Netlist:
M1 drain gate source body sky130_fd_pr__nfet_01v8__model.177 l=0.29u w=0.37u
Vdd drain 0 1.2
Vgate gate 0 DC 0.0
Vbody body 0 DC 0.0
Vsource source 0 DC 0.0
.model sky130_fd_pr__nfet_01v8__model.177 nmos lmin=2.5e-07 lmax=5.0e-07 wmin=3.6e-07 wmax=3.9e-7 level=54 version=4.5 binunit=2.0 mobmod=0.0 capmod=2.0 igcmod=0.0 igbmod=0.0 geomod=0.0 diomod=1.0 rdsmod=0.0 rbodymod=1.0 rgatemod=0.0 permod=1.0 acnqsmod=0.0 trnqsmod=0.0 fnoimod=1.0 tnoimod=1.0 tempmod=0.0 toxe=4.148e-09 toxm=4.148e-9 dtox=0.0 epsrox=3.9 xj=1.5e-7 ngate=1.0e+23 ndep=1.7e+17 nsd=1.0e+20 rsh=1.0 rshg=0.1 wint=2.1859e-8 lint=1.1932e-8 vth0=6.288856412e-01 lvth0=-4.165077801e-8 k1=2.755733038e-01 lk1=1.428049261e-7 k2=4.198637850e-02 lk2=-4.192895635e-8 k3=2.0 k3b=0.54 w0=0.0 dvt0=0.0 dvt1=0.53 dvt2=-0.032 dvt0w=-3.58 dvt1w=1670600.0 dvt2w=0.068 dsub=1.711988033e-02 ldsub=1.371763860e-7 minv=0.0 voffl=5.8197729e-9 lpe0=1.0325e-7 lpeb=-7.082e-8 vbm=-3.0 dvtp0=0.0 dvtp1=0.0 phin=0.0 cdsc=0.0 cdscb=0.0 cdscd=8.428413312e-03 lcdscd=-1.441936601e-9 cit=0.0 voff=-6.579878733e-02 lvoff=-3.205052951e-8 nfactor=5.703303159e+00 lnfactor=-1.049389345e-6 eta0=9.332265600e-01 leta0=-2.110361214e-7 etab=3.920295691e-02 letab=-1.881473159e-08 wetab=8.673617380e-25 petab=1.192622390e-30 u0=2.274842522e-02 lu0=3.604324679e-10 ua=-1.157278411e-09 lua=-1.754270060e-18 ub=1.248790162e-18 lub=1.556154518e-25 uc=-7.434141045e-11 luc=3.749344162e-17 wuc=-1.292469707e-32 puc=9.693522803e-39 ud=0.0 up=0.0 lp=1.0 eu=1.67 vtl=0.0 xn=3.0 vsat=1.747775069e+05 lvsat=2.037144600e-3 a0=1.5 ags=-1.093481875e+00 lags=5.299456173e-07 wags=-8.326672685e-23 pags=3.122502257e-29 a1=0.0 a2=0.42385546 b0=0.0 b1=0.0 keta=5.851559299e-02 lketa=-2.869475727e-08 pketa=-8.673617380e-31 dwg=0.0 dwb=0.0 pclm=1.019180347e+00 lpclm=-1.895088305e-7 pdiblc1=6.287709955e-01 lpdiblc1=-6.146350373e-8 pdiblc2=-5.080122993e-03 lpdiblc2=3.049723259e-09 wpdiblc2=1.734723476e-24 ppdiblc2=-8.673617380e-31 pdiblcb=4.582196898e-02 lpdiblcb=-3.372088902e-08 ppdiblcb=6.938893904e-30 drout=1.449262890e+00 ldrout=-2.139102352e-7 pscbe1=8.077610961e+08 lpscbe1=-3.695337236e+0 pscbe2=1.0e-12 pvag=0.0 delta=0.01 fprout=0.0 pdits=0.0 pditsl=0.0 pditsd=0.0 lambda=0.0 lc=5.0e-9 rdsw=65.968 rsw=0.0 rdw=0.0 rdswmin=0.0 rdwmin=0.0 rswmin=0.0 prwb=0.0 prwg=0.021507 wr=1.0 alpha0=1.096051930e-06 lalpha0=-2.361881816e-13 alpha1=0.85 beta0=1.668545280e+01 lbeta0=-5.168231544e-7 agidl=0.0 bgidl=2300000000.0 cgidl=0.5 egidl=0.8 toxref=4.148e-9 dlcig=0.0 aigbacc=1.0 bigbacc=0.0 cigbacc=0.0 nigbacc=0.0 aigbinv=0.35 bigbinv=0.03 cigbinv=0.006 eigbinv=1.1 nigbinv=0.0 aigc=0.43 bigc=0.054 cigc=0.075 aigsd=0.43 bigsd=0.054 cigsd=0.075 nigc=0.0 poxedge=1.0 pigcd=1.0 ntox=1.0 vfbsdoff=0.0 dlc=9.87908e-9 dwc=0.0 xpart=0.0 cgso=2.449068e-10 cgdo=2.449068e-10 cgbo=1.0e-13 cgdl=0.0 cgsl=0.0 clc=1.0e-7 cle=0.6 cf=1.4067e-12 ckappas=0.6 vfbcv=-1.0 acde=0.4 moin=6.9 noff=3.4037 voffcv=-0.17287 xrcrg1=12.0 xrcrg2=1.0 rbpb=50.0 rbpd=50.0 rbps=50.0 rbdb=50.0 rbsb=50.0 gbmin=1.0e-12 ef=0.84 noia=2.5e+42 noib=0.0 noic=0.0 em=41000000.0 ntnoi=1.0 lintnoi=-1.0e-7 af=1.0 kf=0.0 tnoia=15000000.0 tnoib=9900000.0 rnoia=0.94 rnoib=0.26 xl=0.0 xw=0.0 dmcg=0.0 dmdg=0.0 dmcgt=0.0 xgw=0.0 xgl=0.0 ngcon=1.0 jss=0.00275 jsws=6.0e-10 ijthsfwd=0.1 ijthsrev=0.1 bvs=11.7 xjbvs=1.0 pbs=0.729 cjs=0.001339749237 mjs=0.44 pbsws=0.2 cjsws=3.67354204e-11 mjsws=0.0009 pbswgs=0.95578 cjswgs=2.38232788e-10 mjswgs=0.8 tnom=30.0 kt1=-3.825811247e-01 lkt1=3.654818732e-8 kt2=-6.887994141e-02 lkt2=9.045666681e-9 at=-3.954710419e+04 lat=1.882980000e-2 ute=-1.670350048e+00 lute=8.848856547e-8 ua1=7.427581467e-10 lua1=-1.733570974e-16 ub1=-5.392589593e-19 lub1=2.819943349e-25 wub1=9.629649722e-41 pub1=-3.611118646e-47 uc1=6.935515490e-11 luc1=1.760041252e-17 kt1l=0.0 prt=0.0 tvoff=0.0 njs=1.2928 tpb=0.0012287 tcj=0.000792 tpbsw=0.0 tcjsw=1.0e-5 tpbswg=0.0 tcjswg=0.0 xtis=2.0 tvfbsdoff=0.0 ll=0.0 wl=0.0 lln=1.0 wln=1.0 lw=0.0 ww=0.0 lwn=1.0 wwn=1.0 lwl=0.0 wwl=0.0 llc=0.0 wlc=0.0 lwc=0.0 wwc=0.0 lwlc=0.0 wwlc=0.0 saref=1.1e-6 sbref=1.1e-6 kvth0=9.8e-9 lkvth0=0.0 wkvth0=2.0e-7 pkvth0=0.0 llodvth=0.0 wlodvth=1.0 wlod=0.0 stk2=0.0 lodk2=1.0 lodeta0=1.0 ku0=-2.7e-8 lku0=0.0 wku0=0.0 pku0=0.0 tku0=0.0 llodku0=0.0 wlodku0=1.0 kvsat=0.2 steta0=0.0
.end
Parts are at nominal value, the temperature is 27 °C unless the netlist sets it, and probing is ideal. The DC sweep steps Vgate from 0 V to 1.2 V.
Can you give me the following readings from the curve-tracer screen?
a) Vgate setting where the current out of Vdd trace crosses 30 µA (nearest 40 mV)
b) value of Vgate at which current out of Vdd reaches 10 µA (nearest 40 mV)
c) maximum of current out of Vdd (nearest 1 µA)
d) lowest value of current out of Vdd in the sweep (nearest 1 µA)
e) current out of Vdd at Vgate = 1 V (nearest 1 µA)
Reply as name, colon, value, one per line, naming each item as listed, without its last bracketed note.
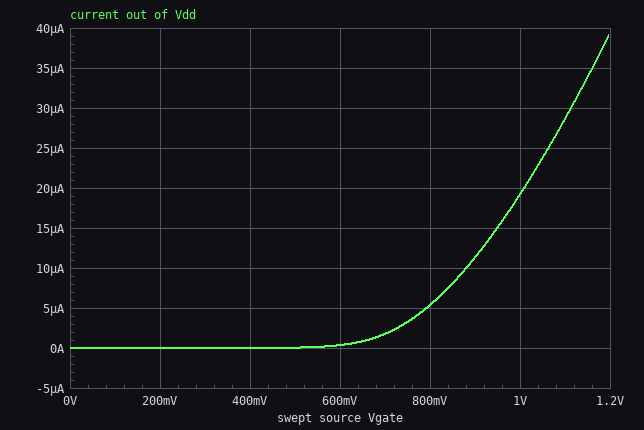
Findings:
Vgate setting where the current out of Vdd trace crosses 30 µA: 1.12 V
value of Vgate at which current out of Vdd reaches 10 µA: 880 mV
maximum of current out of Vdd: 39 µA
lowest value of current out of Vdd in the sweep: 0 A
current out of Vdd at Vgate = 1 V: 19 µA
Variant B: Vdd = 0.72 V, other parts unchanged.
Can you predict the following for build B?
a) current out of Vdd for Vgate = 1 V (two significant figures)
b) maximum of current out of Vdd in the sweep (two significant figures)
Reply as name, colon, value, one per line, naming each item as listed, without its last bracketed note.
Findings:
current out of Vdd for Vgate = 1 V: 18 µA
maximum of current out of Vdd in the sweep: 37 µA
